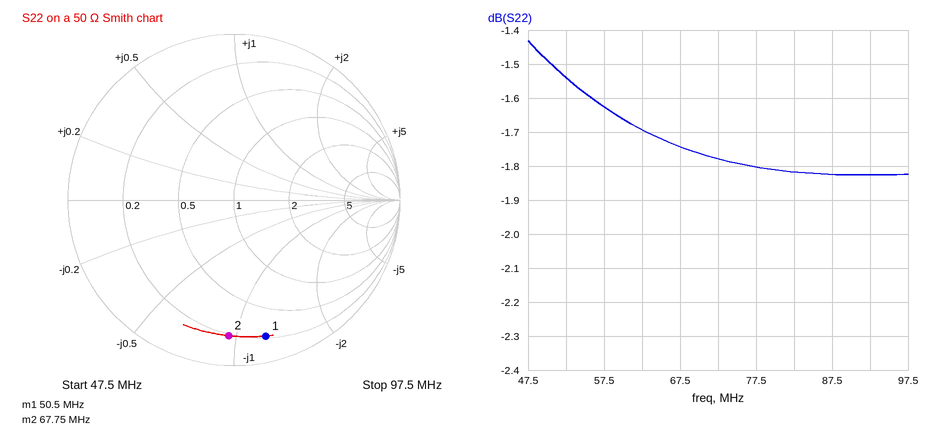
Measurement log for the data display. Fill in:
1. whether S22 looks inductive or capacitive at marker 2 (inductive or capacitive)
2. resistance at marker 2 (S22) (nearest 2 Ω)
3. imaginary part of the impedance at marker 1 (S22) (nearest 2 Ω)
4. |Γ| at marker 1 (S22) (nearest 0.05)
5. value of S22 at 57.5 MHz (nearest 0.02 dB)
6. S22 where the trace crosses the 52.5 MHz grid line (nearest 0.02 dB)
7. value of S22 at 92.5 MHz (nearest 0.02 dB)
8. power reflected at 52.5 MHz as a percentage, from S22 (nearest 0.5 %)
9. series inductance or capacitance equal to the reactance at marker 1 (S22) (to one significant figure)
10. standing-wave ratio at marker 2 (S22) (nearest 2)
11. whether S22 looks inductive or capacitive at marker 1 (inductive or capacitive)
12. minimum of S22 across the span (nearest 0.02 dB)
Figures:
capacitive
10 Ω
-62 Ω
0.85
-1.62 dB
-1.54 dB
-1.82 dB
70.0 %
50 pF
10
capacitive
-1.82 dB
